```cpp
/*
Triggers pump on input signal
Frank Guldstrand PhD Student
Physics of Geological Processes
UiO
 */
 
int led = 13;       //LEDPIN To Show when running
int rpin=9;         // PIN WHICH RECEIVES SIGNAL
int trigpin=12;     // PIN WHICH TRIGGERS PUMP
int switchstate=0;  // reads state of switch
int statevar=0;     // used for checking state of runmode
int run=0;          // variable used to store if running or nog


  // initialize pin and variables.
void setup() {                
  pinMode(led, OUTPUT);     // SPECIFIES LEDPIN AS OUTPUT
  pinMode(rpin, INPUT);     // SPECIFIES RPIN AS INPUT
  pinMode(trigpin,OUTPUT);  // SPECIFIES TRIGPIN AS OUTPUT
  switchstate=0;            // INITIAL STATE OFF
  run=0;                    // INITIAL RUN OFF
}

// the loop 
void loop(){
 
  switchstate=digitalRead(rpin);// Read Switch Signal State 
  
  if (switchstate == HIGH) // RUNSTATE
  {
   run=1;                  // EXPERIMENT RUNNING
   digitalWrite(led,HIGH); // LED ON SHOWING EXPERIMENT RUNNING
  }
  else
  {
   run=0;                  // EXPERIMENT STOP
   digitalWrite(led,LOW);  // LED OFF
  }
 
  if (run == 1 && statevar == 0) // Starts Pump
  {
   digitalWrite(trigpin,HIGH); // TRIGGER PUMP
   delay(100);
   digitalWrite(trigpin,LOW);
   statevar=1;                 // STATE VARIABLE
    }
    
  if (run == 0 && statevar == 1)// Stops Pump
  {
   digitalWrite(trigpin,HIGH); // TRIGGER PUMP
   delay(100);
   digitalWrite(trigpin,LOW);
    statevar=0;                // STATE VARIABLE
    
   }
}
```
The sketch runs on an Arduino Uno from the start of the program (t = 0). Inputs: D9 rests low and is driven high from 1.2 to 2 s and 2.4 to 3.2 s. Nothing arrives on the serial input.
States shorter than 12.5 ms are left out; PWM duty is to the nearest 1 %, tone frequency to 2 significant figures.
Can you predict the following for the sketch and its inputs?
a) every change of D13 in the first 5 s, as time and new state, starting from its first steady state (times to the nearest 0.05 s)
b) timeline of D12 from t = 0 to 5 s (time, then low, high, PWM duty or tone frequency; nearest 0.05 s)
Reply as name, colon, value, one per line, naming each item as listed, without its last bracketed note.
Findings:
every change of D13 in the first 5 s, as time and new state, starting from its first steady state: 0 s low; 1.2 s high; 2 s low; 2.4 s high; 3.2 s low
timeline of D12 from t = 0 to 5 s: 0 s low; 1.2 s high; 1.3 s low; 2 s high; 2.1 s low; 2.4 s high; 2.5 s low; 3.2 s high; 3.3 s low
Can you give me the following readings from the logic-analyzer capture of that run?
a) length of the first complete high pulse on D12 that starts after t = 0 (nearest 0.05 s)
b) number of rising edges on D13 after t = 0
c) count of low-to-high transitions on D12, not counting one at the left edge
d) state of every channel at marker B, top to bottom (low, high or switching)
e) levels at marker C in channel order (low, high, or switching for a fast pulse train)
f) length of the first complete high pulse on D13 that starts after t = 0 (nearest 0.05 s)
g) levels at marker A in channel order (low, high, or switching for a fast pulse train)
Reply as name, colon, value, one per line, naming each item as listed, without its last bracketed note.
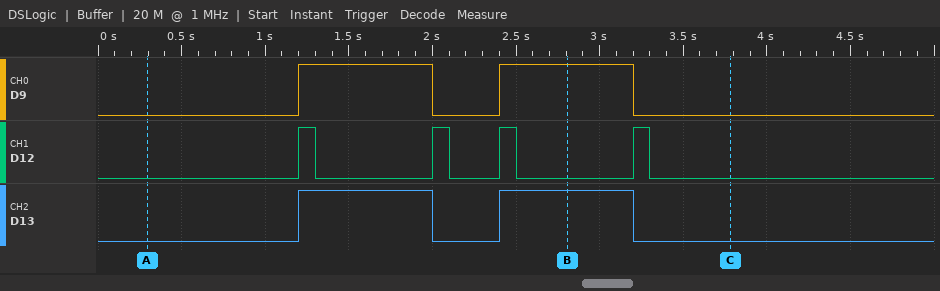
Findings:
length of the first complete high pulse on D12 that starts after t = 0: 0.10 s
number of rising edges on D13 after t = 0: 2
count of low-to-high transitions on D12, not counting one at the left edge: 4
state of every channel at marker B, top to bottom: D9 high, D12 low, D13 high
levels at marker C in channel order: D9 low, D12 low, D13 low
length of the first complete high pulse on D13 that starts after t = 0: 0.80 s
levels at marker A in channel order: D9 low, D12 low, D13 low
